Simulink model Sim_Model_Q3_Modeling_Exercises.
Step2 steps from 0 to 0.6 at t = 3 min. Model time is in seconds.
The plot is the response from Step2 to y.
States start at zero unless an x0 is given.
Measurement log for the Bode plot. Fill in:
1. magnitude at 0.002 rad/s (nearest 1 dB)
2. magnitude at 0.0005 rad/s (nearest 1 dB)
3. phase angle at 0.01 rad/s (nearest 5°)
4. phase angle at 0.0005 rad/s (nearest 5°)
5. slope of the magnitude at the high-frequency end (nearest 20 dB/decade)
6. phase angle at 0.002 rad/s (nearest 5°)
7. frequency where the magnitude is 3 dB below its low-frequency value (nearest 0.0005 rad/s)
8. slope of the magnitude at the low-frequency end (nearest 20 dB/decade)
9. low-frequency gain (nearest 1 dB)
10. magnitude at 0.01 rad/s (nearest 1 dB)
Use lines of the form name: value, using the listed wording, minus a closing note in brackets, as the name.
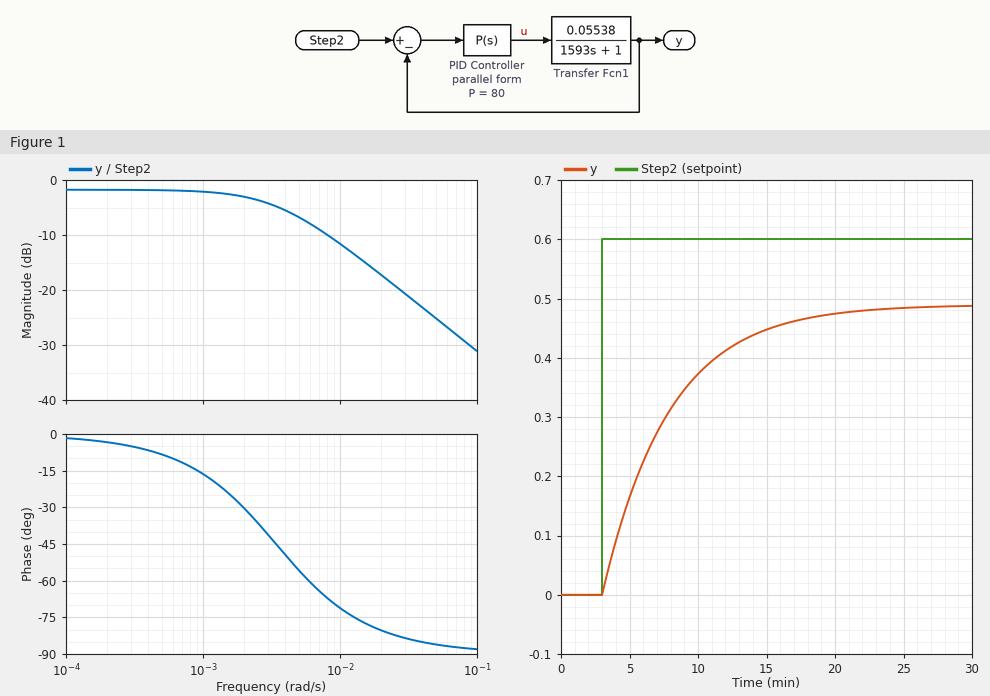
magnitude at 0.002 rad/s: -3 dB
magnitude at 0.0005 rad/s: -2 dB
phase angle at 0.01 rad/s: -70°
phase angle at 0.0005 rad/s: -10°
slope of the magnitude at the high-frequency end: -20 dB/decade
phase angle at 0.002 rad/s: -30°
frequency where the magnitude is 3 dB below its low-frequency value: 0.0035 rad/s
slope of the magnitude at the low-frequency end: 0 dB/decade
low-frequency gain: -2 dB
magnitude at 0.01 rad/s: -12 dB
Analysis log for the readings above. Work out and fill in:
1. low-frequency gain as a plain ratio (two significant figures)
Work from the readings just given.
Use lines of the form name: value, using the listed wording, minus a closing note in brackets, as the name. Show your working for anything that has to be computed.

low-frequency gain as a plain ratio: 10^(-2 / 20) = 0.79
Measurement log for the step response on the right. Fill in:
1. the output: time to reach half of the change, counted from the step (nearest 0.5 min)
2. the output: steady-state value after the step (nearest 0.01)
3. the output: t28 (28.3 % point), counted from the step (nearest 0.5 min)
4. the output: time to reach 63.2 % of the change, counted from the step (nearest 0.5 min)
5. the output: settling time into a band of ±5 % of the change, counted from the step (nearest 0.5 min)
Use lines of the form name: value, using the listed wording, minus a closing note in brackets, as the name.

the output: time to reach half of the change, counted from the step: 3.5 min
the output: steady-state value after the step: 0.49
the output: t28 (28.3 % point), counted from the step: 1.5 min
the output: time to reach 63.2 % of the change, counted from the step: 5.0 min
the output: settling time into a band of ±5 % of the change, counted from the step: 14.5 min
